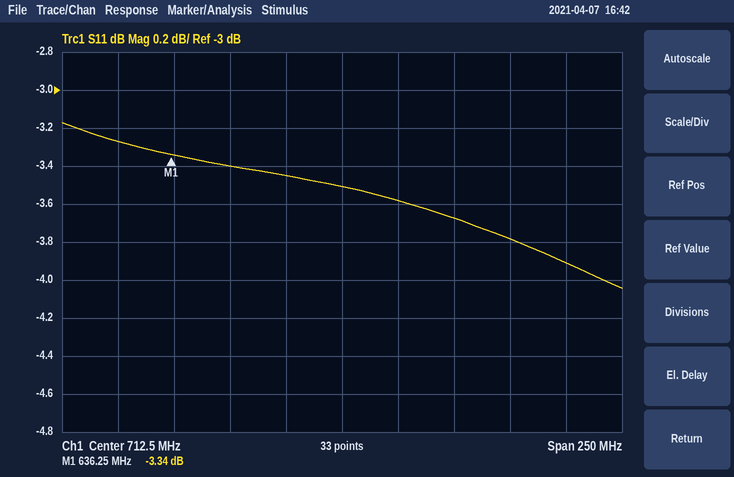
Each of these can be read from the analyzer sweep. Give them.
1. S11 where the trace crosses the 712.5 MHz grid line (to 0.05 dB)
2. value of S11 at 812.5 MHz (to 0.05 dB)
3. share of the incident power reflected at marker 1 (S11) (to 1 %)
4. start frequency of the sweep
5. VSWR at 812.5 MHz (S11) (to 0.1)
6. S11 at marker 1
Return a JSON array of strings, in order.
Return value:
["-3.50 dB", "-3.90 dB", "46 %", "587.5 MHz", "4.5", "-3.34 dB"]
